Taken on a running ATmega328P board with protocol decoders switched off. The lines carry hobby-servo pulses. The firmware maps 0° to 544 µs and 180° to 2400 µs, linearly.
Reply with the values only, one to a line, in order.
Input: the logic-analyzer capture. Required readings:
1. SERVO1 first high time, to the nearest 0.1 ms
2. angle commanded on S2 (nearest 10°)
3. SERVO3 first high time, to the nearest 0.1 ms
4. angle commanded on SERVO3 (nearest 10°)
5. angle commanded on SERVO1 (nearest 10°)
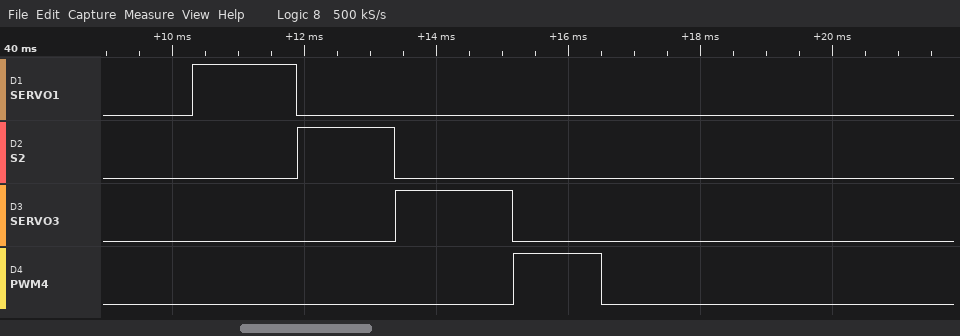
1.6 ms
90°
1.8 ms
120°
100°
